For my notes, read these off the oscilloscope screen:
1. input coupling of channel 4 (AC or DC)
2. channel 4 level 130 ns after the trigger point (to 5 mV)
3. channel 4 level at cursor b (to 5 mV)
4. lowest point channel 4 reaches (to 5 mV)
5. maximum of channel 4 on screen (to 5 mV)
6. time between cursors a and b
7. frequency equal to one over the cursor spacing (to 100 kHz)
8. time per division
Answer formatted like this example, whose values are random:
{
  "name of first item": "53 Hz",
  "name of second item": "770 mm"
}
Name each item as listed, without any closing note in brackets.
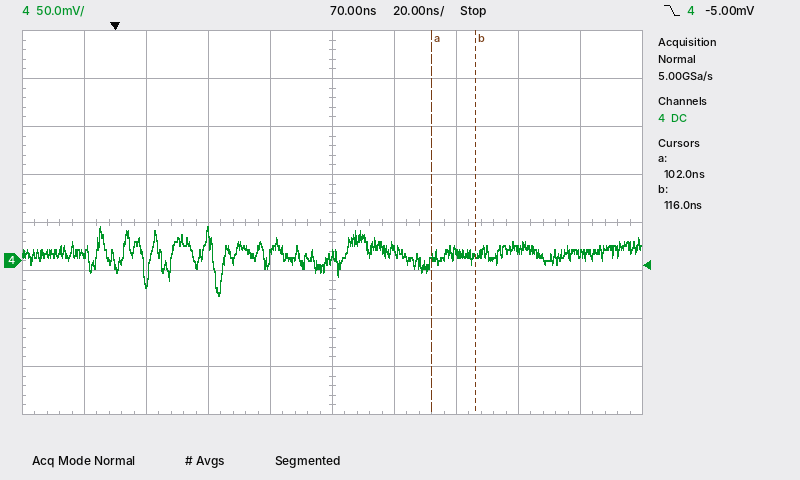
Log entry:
{
  "input coupling of channel 4": "DC",
  "channel 4 level 130 ns after the trigger point": "10 mV",
  "channel 4 level at cursor b": "5 mV",
  "lowest point channel 4 reaches": "-35 mV",
  "maximum of channel 4 on screen": "35 mV",
  "time between cursors a and b": "14 ns",
  "frequency equal to one over the cursor spacing": "71.4 MHz",
  "time per division": "20 ns"
}
